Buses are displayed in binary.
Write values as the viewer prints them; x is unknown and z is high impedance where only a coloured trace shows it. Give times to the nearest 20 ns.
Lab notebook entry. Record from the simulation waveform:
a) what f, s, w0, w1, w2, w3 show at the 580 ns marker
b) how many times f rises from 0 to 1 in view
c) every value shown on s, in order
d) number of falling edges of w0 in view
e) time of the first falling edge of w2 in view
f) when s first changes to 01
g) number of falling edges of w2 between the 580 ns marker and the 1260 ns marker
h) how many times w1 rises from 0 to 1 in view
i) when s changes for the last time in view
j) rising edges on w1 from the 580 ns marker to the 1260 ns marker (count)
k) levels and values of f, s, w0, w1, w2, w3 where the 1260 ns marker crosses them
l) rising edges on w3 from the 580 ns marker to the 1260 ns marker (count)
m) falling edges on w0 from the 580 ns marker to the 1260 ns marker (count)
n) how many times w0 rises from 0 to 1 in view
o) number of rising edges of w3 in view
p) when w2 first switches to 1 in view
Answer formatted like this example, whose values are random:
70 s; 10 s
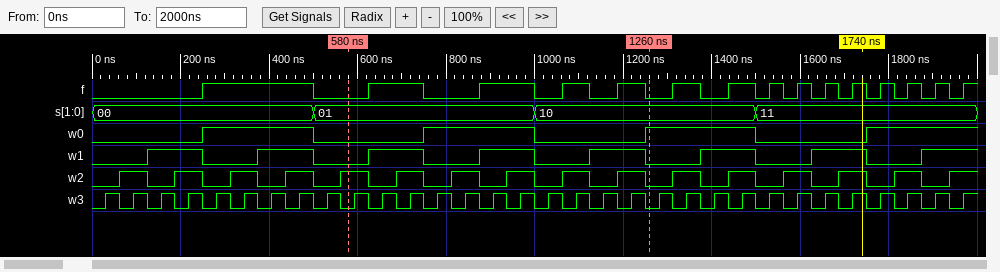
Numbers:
f=0, s=01, w0=0, w1=0, w2=1, w3=0; 15; 00, 01, 10, 11; 3; 120 ns; 500 ns; 6; 8; 1500 ns; 3; f=0, s=10, w0=1, w1=0, w2=0, w3=0; 11; 1; 4; 32; 60 ns
